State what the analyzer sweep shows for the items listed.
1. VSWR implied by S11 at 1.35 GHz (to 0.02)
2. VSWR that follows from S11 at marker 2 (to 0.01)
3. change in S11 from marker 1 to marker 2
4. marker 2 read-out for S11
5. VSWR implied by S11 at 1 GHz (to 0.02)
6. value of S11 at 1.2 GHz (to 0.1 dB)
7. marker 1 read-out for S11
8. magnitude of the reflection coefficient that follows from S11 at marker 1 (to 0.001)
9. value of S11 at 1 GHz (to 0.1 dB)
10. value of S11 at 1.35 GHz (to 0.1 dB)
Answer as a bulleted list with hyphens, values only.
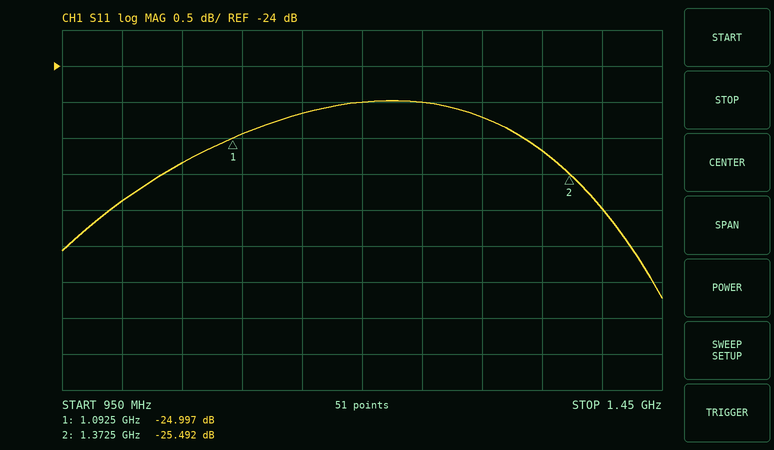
- 1.12
- 1.11
- -0.495 dB
- -25.492 dB
- 1.10
- -24.5 dB
- -24.997 dB
- 0.056
- -25.9 dB
- -25.2 dB
